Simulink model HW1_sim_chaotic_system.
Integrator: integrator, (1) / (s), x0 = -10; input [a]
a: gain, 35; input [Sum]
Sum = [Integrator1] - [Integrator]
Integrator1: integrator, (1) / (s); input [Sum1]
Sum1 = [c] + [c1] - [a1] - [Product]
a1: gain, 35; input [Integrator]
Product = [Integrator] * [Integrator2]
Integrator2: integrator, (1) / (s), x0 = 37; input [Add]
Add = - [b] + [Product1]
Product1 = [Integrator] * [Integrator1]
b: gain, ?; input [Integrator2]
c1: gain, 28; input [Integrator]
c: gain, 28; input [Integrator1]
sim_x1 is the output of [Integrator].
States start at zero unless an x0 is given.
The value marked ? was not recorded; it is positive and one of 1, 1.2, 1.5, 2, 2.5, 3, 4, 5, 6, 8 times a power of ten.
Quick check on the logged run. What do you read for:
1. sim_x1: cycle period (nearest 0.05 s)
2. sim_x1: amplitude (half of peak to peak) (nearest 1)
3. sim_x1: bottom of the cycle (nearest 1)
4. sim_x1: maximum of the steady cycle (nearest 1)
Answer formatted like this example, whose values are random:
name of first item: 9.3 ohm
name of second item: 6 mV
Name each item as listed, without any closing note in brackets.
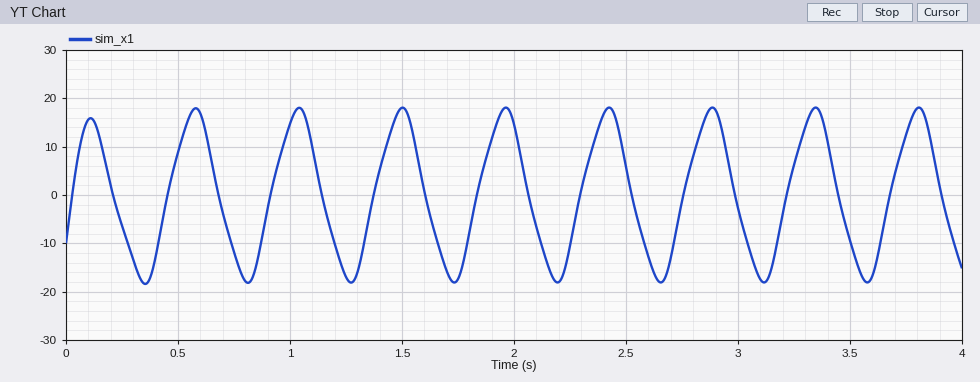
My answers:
sim_x1: cycle period: 0.45 s
sim_x1: amplitude (half of peak to peak): 18
sim_x1: bottom of the cycle: -18
sim_x1: maximum of the steady cycle: 18
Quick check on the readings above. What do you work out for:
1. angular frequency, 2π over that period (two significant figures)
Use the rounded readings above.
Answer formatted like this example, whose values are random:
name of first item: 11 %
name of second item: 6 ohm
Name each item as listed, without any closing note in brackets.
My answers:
angular frequency, 2π over that period: 14 rad/s
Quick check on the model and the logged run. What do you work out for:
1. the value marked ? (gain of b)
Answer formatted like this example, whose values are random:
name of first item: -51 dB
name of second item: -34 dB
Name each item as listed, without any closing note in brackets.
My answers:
the value marked ?: 6
